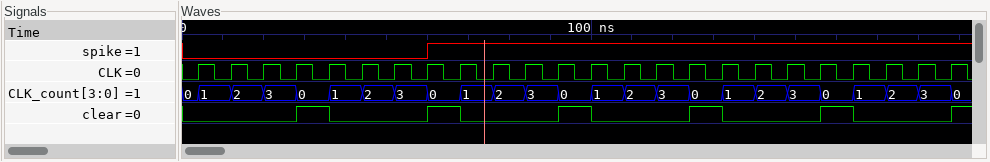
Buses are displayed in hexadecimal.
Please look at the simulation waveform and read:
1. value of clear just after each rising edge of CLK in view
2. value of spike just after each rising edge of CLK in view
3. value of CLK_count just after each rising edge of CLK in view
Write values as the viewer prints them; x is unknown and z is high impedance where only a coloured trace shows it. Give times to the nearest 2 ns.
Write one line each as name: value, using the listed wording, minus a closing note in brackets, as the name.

value of clear just after each rising edge of CLK in view: 0 0 0 1 0 0 0 1 0 0 0 1 0 0 0 1 0 0 0 1 0 0 0 1
value of spike just after each rising edge of CLK in view: 0 0 0 0 0 0 0 1 1 1 1 1 1 1 1 1 1 1 1 1 1 1 1 1
value of CLK_count just after each rising edge of CLK in view: 1, 2, 3, 0, 1, 2, 3, 0, 1, 2, 3, 0, 1, 2, 3, 0, 1, 2, 3, 0, 1, 2, 3, 0
